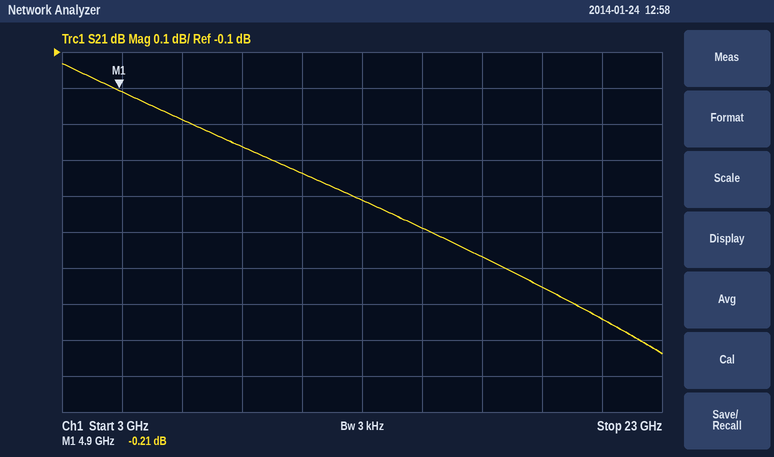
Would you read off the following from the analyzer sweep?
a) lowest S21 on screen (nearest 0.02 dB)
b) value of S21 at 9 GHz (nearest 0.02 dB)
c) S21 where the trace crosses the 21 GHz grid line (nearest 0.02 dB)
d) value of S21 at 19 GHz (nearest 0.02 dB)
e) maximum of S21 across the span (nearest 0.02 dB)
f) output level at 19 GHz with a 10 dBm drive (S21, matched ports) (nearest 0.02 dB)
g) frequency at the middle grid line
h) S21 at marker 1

-0.94 dB
-0.36 dB
-0.84 dB
-0.76 dB
-0.14 dB
9.24 dBm
13 GHz
-0.21 dB
